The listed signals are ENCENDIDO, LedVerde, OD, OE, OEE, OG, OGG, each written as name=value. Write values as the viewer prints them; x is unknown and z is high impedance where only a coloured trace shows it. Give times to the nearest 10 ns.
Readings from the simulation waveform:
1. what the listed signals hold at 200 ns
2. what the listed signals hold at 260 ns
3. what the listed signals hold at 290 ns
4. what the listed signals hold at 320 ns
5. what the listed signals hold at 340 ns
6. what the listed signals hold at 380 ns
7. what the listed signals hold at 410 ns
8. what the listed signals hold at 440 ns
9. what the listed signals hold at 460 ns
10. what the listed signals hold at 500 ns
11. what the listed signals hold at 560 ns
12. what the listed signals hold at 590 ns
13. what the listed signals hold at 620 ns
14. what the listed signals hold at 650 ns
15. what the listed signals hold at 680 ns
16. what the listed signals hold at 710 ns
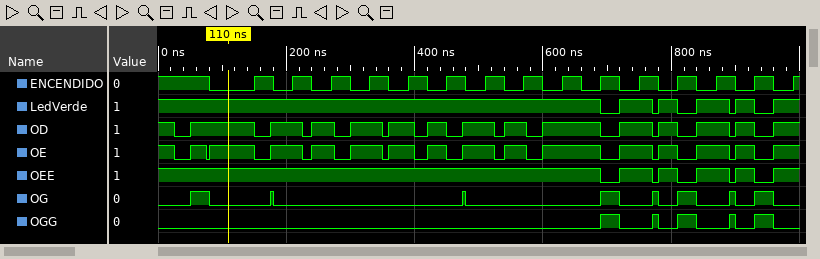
ENCENDIDO=0, LedVerde=1, OD=1, OE=1, OEE=1, OG=0, OGG=0
ENCENDIDO=0, LedVerde=1, OD=1, OE=1, OEE=1, OG=0, OGG=0
ENCENDIDO=1, LedVerde=1, OD=0, OE=0, OEE=1, OG=0, OGG=0
ENCENDIDO=0, LedVerde=1, OD=1, OE=1, OEE=1, OG=0, OGG=0
ENCENDIDO=1, LedVerde=1, OD=1, OE=1, OEE=1, OG=0, OGG=0
ENCENDIDO=0, LedVerde=1, OD=1, OE=1, OEE=1, OG=0, OGG=0
ENCENDIDO=1, LedVerde=1, OD=0, OE=0, OEE=1, OG=0, OGG=0
ENCENDIDO=0, LedVerde=1, OD=1, OE=1, OEE=1, OG=0, OGG=0
ENCENDIDO=1, LedVerde=1, OD=0, OE=0, OEE=1, OG=0, OGG=0
ENCENDIDO=0, LedVerde=1, OD=1, OE=1, OEE=1, OG=0, OGG=0
ENCENDIDO=0, LedVerde=1, OD=1, OE=1, OEE=1, OG=0, OGG=0
ENCENDIDO=1, LedVerde=1, OD=0, OE=0, OEE=1, OG=0, OGG=0
ENCENDIDO=0, LedVerde=1, OD=1, OE=1, OEE=1, OG=0, OGG=0
ENCENDIDO=1, LedVerde=1, OD=1, OE=1, OEE=1, OG=0, OGG=0
ENCENDIDO=0, LedVerde=1, OD=1, OE=1, OEE=1, OG=0, OGG=0
ENCENDIDO=1, LedVerde=0, OD=0, OE=0, OEE=0, OG=1, OGG=1
